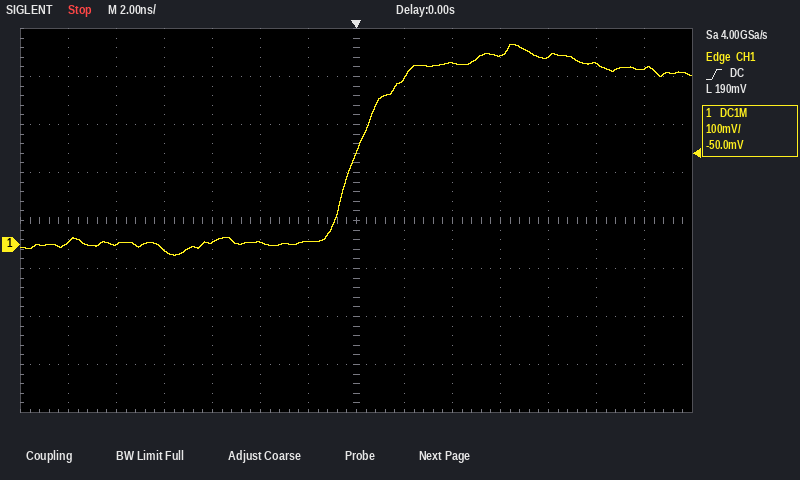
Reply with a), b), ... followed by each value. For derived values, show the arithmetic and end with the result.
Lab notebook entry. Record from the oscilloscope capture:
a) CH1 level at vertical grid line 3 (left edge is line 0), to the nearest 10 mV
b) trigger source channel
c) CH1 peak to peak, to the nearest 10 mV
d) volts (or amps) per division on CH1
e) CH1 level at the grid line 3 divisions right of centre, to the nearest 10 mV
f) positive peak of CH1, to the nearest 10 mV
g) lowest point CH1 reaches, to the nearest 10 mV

a) -10 mV
b) CH1
c) 420 mV − (-20 mV) = 440 mV
d) 100 mV
e) 390 mV
f) 420 mV
g) -20 mV
